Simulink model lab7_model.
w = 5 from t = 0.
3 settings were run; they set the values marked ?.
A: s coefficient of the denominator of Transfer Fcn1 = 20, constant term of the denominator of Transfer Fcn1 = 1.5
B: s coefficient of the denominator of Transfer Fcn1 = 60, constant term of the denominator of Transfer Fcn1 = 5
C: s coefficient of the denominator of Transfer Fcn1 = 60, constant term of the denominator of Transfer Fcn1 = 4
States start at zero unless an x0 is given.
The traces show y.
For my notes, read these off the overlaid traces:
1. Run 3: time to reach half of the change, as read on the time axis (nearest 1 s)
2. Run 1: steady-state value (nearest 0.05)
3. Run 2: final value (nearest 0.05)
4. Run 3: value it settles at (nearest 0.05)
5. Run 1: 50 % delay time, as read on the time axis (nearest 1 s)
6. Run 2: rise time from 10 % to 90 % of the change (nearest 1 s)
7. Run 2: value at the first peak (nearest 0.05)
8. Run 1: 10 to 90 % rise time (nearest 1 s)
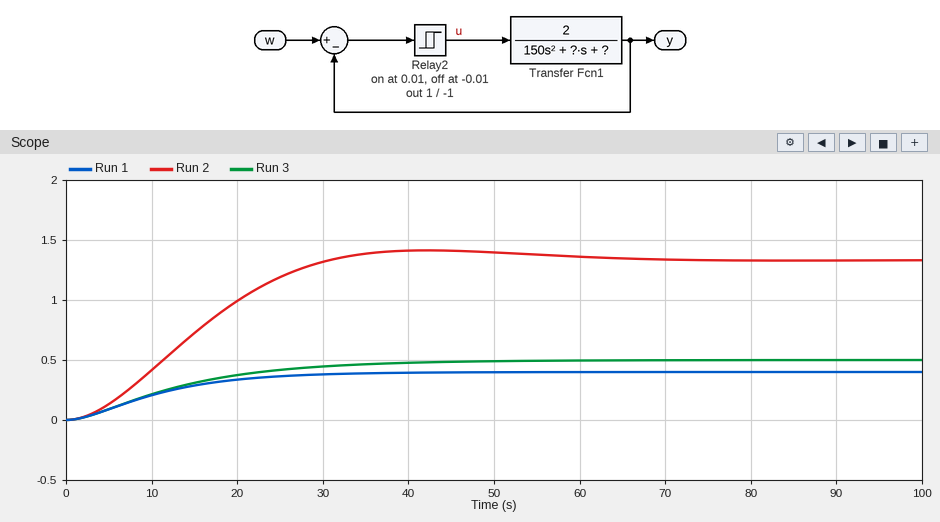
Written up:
12 s
0.40
1.35
0.50
10 s
20 s
1.40
21 s
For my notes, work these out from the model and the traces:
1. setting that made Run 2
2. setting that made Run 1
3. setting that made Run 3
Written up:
A
B
C
